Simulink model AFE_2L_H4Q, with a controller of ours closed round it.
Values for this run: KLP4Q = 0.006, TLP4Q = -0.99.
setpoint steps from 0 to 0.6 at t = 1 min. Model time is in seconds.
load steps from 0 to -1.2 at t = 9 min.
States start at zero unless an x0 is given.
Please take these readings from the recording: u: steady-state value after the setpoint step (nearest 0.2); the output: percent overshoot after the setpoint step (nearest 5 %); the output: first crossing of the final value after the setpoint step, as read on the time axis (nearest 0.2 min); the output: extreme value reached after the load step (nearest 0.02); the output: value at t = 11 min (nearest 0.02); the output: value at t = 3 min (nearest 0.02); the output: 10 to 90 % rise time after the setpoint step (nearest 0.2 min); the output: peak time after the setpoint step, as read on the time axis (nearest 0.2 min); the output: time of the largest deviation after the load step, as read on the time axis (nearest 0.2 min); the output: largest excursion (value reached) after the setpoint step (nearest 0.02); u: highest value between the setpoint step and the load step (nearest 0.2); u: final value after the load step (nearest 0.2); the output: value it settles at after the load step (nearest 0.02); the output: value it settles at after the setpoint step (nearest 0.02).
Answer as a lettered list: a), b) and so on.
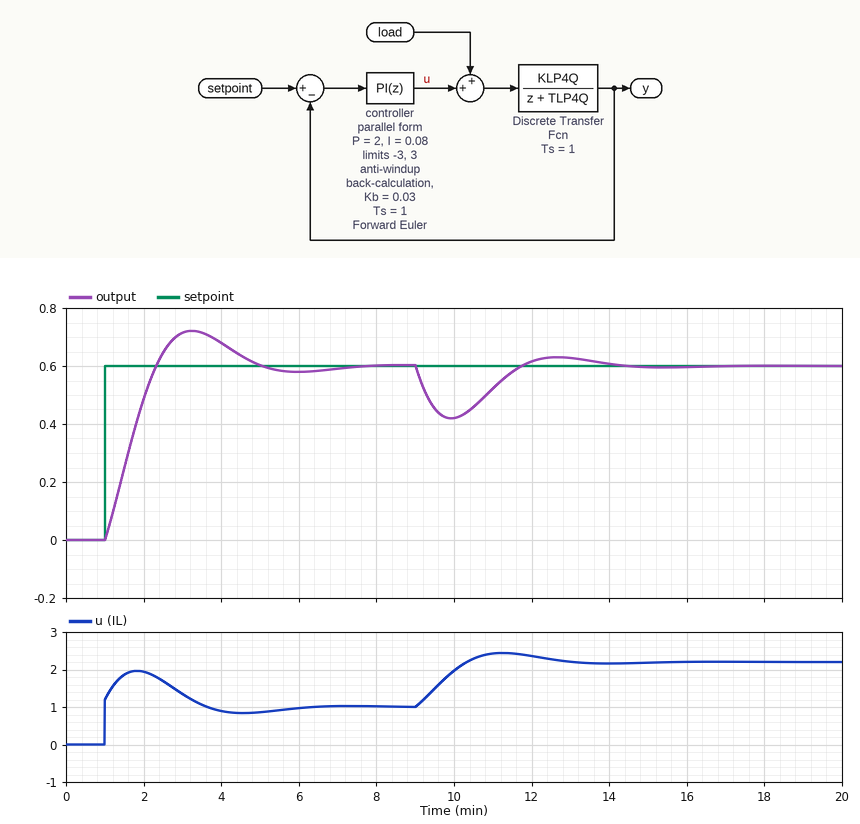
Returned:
a) 1.0
b) 20 %
c) 2.4 min
d) 0.42
e) 0.52
f) 0.72
g) 1.0 min
h) 3.2 min
i) 10.0 min
j) 0.72
k) 2.0
l) 2.2
m) 0.60
n) 0.60
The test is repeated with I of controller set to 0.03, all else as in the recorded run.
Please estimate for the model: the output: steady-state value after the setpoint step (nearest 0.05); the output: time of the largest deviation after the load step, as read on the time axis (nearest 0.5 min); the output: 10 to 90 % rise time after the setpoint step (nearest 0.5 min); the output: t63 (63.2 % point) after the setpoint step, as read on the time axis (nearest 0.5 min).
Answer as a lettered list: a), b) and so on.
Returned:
a) 0.60
b) 10.5 min
c) 2.0 min
d) 2.0 min
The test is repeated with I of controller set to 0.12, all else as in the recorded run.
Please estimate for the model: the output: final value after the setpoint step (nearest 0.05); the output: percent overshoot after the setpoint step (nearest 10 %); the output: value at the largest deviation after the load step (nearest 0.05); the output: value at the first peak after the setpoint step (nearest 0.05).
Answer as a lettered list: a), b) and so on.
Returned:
a) 0.60
b) 30 %
c) 0.45
d) 0.75
